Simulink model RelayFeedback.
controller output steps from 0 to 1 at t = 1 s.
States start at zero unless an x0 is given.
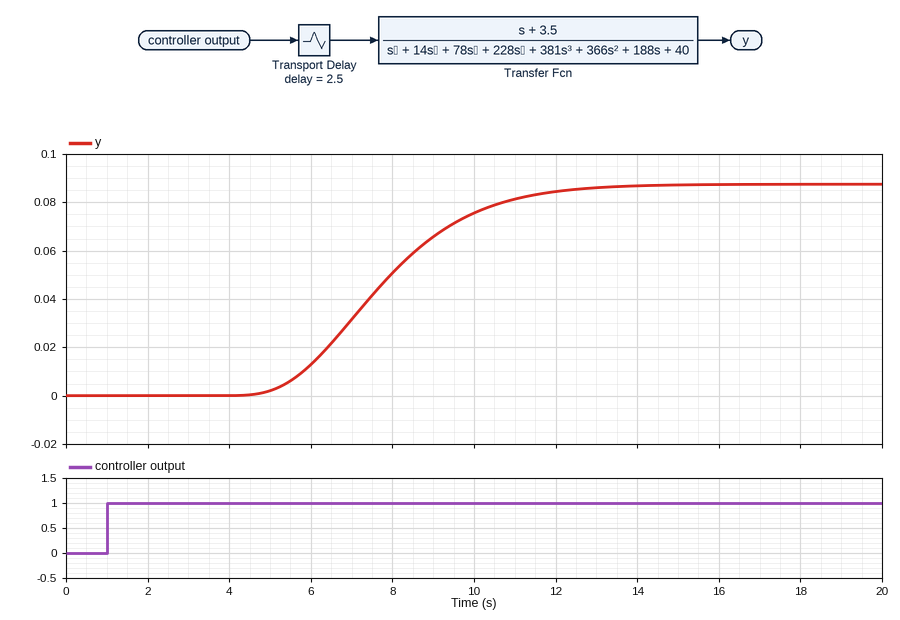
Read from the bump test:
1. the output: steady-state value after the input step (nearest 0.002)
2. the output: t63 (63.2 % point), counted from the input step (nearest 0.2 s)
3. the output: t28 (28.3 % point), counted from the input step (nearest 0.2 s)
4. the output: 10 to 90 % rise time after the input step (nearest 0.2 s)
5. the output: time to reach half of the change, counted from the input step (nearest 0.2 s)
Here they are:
0.088
7.2 s
5.6 s
4.8 s
6.6 s
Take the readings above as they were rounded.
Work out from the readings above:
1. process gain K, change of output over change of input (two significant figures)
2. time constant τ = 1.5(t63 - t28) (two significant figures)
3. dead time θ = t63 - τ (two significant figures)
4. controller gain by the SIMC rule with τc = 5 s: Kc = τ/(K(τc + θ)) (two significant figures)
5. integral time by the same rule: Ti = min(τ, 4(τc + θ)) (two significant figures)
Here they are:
0.088
2.4 s
4.8 s
2.8
2.4 s
